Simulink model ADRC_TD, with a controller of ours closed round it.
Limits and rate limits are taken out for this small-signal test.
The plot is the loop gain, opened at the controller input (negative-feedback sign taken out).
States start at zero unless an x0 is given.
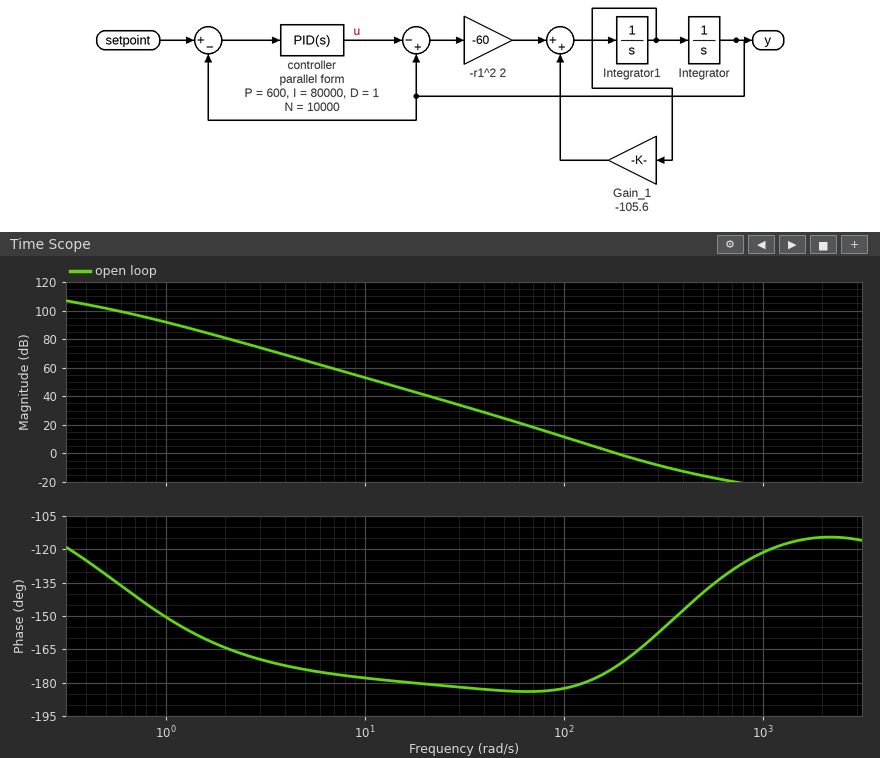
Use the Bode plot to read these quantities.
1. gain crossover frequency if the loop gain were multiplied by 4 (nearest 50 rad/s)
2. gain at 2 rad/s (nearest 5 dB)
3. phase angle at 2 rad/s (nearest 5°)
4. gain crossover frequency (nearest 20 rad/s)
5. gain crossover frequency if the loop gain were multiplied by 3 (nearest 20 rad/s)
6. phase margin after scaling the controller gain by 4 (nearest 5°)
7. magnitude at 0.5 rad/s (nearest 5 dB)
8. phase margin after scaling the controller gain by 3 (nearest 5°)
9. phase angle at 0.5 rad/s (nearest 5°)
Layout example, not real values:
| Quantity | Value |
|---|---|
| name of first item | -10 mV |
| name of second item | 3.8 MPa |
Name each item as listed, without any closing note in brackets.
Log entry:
| Quantity | Value |
|---|---|
| gain crossover frequency if the loop gain were multiplied by 4 | 400 rad/s |
| gain at 2 rad/s | 80 dB |
| phase angle at 2 rad/s | -165° |
| gain crossover frequency | 180 rad/s |
| gain crossover frequency if the loop gain were multiplied by 3 | 320 rad/s |
| phase margin after scaling the controller gain by 4 | 30° |
| magnitude at 0.5 rad/s | 100 dB |
| phase margin after scaling the controller gain by 3 | 25° |
| phase angle at 0.5 rad/s | -130° |
